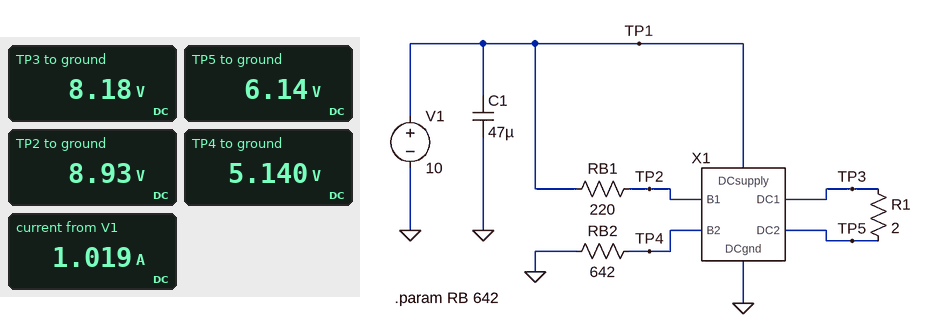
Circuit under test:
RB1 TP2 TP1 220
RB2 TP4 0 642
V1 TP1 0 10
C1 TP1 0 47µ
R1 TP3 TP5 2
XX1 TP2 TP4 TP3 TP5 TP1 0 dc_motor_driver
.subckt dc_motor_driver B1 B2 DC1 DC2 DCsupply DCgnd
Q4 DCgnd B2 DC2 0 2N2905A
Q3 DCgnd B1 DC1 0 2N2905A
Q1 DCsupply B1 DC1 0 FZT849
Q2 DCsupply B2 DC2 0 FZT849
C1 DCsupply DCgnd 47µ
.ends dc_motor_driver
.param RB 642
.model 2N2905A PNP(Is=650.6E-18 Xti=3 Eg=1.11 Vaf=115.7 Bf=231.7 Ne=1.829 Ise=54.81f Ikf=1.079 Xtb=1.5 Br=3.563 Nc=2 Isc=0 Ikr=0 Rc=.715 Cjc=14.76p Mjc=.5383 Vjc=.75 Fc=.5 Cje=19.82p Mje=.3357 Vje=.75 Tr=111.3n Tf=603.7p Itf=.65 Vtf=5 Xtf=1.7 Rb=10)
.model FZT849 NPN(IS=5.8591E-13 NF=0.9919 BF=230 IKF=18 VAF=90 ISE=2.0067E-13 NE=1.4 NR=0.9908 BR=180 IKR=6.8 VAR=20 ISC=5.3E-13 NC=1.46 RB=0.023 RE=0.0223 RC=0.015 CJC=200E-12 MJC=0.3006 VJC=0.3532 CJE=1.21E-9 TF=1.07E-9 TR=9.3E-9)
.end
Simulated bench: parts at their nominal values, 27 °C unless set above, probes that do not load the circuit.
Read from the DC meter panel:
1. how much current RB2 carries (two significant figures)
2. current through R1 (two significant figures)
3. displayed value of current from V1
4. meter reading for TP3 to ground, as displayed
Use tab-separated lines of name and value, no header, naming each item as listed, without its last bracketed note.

how much current RB2 carries	8.0 mA
current through R1	1.0 A
displayed value of current from V1	1.019 A
meter reading for TP3 to ground, as displayed	8.18 V
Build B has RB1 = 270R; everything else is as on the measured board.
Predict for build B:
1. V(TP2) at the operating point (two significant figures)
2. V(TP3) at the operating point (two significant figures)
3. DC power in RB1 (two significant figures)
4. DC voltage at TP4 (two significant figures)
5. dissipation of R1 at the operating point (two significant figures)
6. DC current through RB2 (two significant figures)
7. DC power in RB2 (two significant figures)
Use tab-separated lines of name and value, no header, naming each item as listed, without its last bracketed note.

V(TP2) at the operating point	8.7 V
V(TP3) at the operating point	8.0 V
DC power in RB1	6.1 mW
DC voltage at TP4	5.0 V
dissipation of R1 at the operating point	2.0 W
DC current through RB2	7.8 mA
DC power in RB2	39 mW
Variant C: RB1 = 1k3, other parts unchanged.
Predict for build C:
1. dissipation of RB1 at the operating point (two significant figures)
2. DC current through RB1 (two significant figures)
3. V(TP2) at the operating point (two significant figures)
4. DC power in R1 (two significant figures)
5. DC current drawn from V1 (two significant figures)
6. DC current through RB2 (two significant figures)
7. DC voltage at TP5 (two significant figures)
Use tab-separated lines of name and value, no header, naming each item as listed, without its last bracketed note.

dissipation of RB1 at the operating point	12 mW
DC current through RB1	3.1 mA
V(TP2) at the operating point	6.0 V
DC power in R1	920 mW
DC current drawn from V1	680 mA
DC current through RB2	4.6 mA
DC voltage at TP5	3.9 V
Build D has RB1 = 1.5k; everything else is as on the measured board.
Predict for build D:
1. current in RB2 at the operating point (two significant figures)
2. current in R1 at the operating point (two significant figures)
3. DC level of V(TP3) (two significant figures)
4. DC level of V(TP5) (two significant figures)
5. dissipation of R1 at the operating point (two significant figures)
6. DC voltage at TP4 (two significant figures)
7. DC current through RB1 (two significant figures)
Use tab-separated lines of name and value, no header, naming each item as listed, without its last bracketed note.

current in RB2 at the operating point	4.2 mA
current in R1 at the operating point	640 mA
DC level of V(TP3)	4.9 V
DC level of V(TP5)	3.7 V
dissipation of R1 at the operating point	810 mW
DC voltage at TP4	2.7 V
DC current through RB1	2.9 mA
